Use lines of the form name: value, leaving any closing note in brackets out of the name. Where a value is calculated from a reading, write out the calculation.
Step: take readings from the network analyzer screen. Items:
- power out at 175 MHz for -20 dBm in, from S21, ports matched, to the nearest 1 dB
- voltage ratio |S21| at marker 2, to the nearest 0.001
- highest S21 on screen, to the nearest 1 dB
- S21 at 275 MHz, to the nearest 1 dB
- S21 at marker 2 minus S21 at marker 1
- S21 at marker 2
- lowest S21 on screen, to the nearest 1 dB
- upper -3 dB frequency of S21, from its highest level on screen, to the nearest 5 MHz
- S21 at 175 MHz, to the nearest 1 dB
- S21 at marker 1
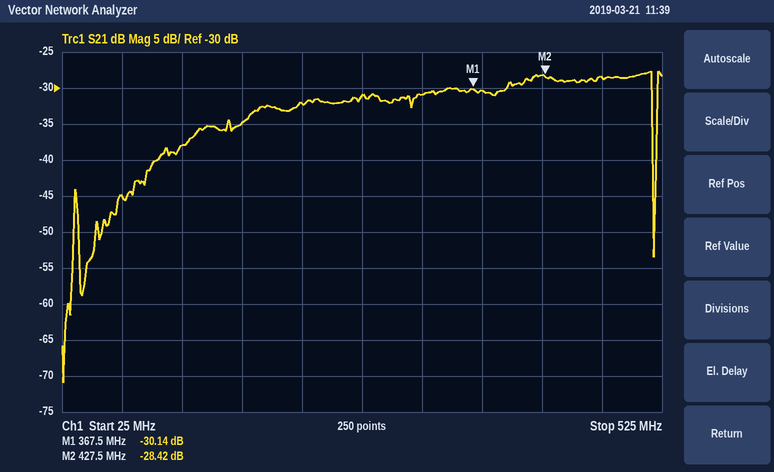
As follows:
power out at 175 MHz for -20 dBm in, from S21, ports matched, to the nearest 1 dB: -20 dBm + (-35 dB) = -55 dBm
voltage ratio |S21| at marker 2, to the nearest 0.001: 10^(-28.42/20) ≈ 0.038
highest S21 on screen, to the nearest 1 dB: -28 dB
S21 at 275 MHz, to the nearest 1 dB: -31 dB
S21 at marker 2 minus S21 at marker 1: -28.42 − (-30.14) = 1.72 dB
S21 at marker 2: -28.42 dB
lowest S21 on screen, to the nearest 1 dB: -71 dB
upper -3 dB frequency of S21, from its highest level on screen, to the nearest 5 MHz: 515 MHz
S21 at 175 MHz, to the nearest 1 dB: -35 dB
S21 at marker 1: -30.14 dB
